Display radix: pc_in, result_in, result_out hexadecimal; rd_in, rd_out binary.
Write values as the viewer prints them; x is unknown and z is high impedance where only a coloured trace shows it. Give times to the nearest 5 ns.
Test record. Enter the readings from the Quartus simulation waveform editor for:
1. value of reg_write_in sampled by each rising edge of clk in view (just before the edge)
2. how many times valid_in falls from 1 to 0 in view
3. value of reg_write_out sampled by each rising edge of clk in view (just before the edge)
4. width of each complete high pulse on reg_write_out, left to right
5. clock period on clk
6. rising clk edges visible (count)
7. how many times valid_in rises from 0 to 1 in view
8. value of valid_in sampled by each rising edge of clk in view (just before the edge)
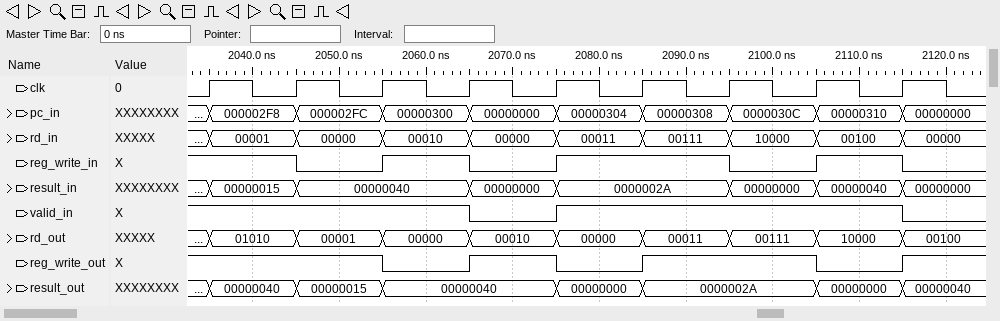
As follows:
1 1 0 1 0 1 1 0 1
2
1 1 1 0 1 0 1 1 0
10 ns, 20 ns
10 ns
9
1
1 1 1 1 0 1 1 1 1
